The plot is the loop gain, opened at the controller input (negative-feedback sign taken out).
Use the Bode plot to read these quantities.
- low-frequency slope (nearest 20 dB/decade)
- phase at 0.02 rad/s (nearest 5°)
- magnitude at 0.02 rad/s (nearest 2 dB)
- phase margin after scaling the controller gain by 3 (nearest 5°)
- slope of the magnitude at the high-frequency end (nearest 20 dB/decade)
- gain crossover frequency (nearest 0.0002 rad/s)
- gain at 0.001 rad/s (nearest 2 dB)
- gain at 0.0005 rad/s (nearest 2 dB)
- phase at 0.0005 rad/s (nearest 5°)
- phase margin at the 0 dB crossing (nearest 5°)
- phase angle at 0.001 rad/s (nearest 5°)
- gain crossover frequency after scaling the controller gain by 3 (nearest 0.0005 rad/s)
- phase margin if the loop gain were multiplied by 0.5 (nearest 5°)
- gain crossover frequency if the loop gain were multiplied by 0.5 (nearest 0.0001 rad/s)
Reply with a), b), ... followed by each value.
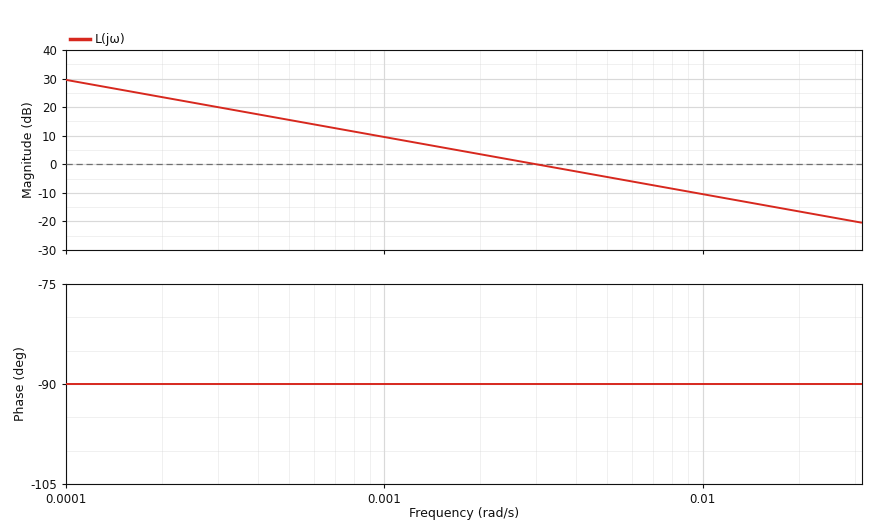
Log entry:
a) -20 dB/decade
b) -90°
c) -16 dB
d) 90°
e) -20 dB/decade
f) 0.0030 rad/s
g) 10 dB
h) 16 dB
i) -90°
j) 90°
k) -90°
l) 0.0090 rad/s
m) 90°
n) 0.0015 rad/s
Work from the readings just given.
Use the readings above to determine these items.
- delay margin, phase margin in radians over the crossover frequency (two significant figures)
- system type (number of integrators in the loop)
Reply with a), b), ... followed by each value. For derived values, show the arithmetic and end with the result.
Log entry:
a) 90 × π / 180 / 0.003 = 520 s
b) 1
